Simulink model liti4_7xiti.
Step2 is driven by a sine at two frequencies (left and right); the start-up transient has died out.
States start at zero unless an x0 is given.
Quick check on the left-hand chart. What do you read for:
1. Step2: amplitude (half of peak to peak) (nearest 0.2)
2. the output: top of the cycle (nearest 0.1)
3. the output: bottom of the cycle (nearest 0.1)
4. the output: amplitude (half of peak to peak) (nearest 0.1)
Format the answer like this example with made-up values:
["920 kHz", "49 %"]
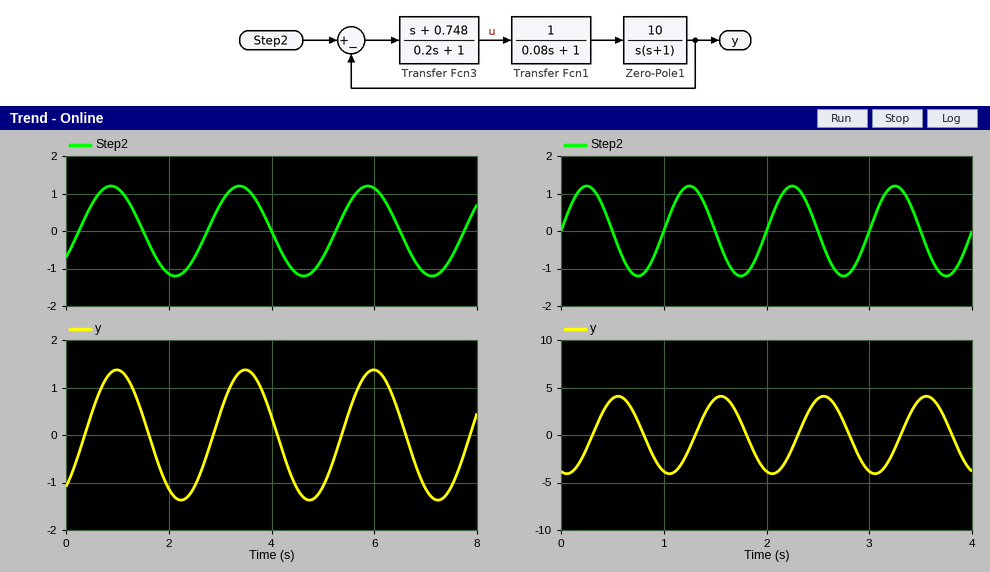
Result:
["1.2", "1.4", "-1.4", "1.4"]
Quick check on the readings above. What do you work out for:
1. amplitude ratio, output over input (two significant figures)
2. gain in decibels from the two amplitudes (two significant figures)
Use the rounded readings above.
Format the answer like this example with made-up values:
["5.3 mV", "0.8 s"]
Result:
["1.2", "1.3 dB"]
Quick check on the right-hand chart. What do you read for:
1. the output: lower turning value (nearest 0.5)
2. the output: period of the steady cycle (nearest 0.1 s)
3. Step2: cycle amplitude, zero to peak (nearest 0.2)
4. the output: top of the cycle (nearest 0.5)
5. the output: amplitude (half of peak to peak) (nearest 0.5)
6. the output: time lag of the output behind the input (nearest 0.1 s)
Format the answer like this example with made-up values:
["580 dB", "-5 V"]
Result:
["-4.0", "1.0 s", "1.2", "4.0", "4.0", "0.3 s"]
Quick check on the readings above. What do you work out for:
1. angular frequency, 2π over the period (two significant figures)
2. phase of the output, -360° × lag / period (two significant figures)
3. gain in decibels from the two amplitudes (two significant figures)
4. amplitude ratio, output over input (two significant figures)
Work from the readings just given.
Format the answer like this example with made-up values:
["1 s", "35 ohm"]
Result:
["6.3 rad/s", "-110°", "10 dB", "3.3"]
